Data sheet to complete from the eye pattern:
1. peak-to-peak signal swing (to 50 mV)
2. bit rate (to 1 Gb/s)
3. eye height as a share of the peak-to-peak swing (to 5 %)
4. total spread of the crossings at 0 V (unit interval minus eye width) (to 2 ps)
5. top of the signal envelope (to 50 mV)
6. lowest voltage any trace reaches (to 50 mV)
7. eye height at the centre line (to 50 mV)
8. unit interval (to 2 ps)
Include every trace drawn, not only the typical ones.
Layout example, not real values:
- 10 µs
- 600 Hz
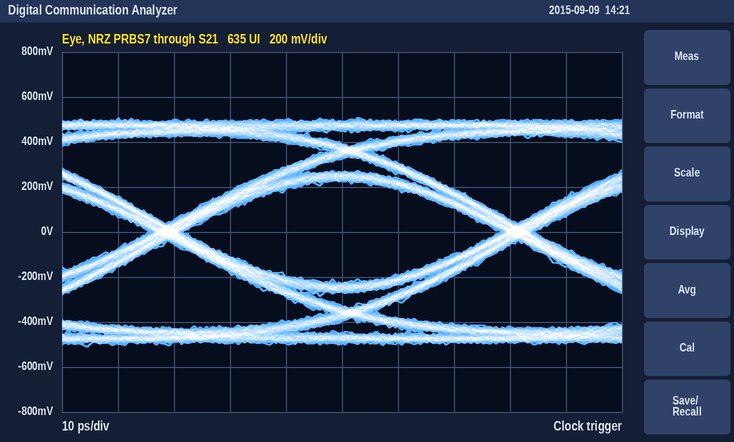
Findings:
- 1.00 V
- 16 Gb/s
- 45 %
- 6 ps
- 500 mV
- -500 mV
- 450 mV
- 62 ps
